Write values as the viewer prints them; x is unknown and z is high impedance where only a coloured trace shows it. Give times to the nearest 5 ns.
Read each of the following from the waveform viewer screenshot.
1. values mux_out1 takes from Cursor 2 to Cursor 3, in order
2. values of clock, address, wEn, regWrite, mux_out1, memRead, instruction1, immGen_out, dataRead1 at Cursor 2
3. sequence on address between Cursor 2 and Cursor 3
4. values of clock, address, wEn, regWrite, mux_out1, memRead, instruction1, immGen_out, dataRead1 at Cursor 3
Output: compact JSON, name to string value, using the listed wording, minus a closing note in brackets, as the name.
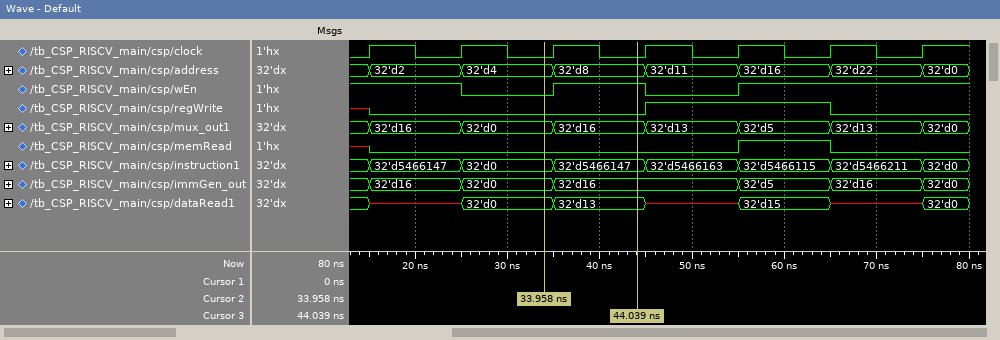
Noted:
{"values mux_out1 takes from Cursor 2 to Cursor 3, in order": "32'd0, 32'd16", "values of clock, address, wEn, regWrite, mux_out1, memRead, instruction1, immGen_out, dataRead1 at Cursor 2": "clock=0, address=32'd4, wEn=0, regWrite=0, mux_out1=32'd0, memRead=0, instruction1=32'd0, immGen_out=32'd0, dataRead1=32'd0", "sequence on address between Cursor 2 and Cursor 3": "32'd4, 32'd8", "values of clock, address, wEn, regWrite, mux_out1, memRead, instruction1, immGen_out, dataRead1 at Cursor 3": "clock=0, address=32'd8, wEn=1, regWrite=0, mux_out1=32'd16, memRead=0, instruction1=32'd5466147, immGen_out=32'd16, dataRead1=32'd13"}
